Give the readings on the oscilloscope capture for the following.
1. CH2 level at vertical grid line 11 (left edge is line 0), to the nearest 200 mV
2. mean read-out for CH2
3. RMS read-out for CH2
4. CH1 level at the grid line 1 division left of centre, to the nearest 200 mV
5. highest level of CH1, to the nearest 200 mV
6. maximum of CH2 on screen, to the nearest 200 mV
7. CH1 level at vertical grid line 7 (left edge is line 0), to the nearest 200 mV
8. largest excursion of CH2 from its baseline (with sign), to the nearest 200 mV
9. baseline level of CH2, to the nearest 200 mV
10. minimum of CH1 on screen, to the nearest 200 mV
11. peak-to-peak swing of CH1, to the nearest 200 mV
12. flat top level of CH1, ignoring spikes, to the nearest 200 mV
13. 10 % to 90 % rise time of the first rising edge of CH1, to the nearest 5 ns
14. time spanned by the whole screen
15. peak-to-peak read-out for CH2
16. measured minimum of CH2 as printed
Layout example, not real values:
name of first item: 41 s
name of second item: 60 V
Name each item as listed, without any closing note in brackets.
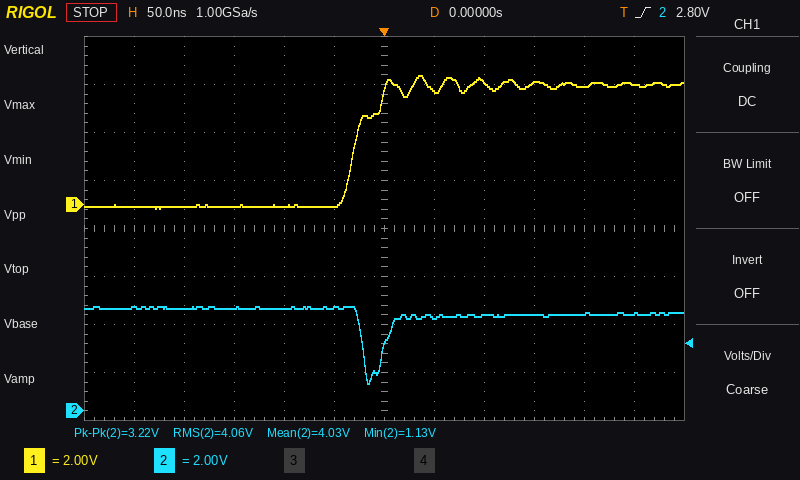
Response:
CH2 level at vertical grid line 11 (left edge is line 0), to the nearest 200 mV: 4.0 V
mean read-out for CH2: 4.03 V
RMS read-out for CH2: 4.06 V
CH1 level at the grid line 1 division left of centre, to the nearest 200 mV: 0.0 V
highest level of CH1, to the nearest 200 mV: 5.4 V
maximum of CH2 on screen, to the nearest 200 mV: 4.4 V
CH1 level at vertical grid line 7 (left edge is line 0), to the nearest 200 mV: 4.8 V
largest excursion of CH2 from its baseline (with sign), to the nearest 200 mV: -3.0 V
baseline level of CH2, to the nearest 200 mV: 4.0 V
minimum of CH1 on screen, to the nearest 200 mV: -200 mV
peak-to-peak swing of CH1, to the nearest 200 mV: 5.6 V
flat top level of CH1, ignoring spikes, to the nearest 200 mV: 5.0 V
10 % to 90 % rise time of the first rising edge of CH1, to the nearest 5 ns: 40 ns
time spanned by the whole screen: 600 ns
peak-to-peak read-out for CH2: 3.22 V
measured minimum of CH2 as printed: 1.13 V
